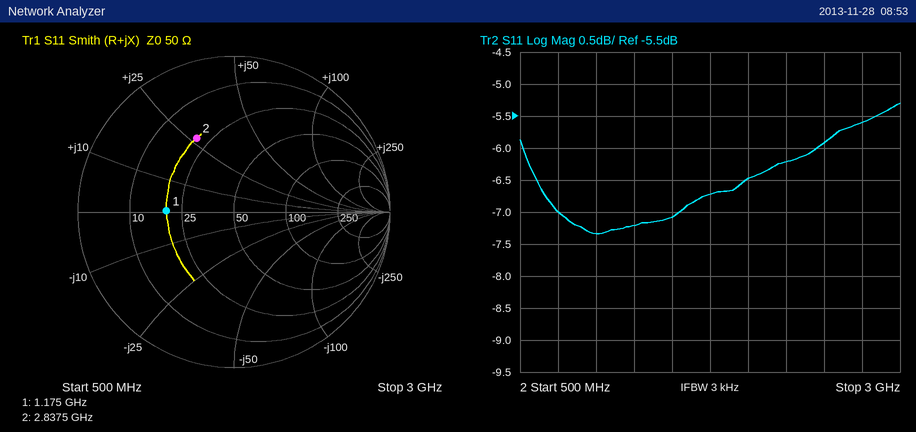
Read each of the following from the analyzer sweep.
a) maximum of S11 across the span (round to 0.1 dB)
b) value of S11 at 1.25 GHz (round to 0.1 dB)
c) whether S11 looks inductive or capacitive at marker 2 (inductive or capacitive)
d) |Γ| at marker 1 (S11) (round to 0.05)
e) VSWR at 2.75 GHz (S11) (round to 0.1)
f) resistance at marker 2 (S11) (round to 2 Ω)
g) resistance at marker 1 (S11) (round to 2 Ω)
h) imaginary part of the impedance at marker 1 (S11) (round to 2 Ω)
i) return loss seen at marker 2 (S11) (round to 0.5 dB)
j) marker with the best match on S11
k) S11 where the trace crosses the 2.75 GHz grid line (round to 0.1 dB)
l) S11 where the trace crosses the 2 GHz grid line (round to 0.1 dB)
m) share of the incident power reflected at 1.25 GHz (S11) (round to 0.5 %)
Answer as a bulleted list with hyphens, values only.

- -5.3 dB
- -7.2 dB
- inductive
- 0.45
- 3.2
- 20 Ω
- 20 Ω
- 0 Ω
- 5.5 dB
- marker 1
- -5.6 dB
- -6.5 dB
- 19.0 %
